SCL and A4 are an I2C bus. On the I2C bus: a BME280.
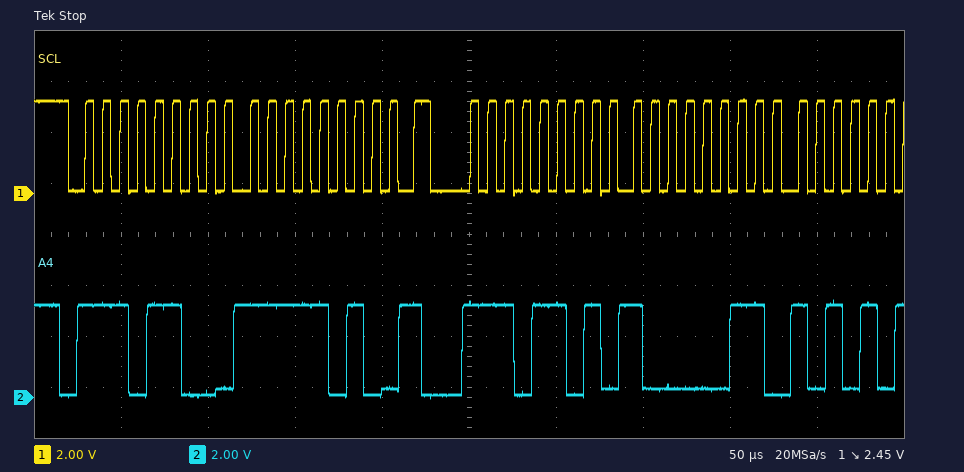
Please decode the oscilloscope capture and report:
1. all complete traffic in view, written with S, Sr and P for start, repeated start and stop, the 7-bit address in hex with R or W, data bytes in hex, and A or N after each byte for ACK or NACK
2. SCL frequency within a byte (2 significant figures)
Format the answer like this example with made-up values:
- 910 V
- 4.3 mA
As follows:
- S 76W A FA A Sr 76R A 83 A
- 100 kHz
